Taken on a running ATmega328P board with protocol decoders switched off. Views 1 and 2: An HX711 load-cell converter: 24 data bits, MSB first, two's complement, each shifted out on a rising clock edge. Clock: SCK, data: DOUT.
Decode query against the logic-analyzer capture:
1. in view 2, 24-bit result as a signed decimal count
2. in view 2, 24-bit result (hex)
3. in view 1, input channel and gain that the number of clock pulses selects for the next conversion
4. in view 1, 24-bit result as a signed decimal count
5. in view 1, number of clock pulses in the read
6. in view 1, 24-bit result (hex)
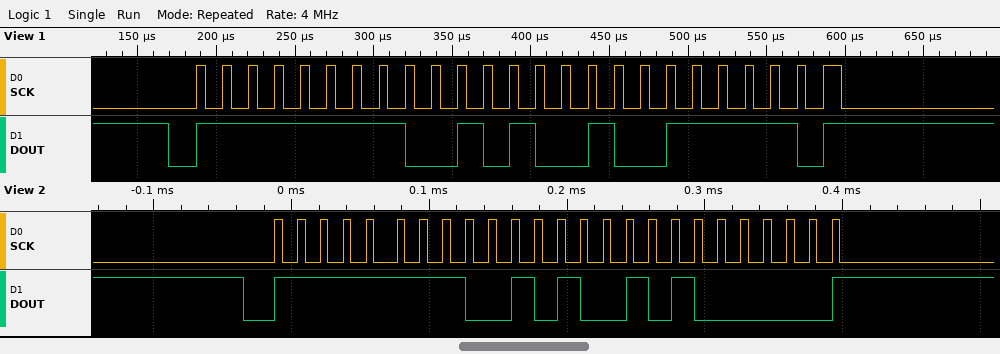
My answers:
-54976
0xFF2940
channel A, gain 128
-54978
25
0xFF293E
